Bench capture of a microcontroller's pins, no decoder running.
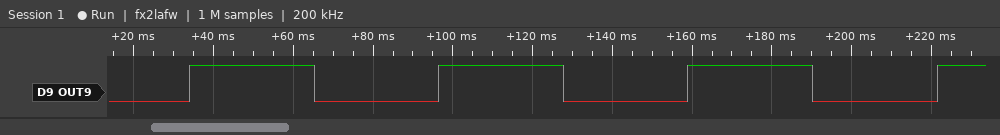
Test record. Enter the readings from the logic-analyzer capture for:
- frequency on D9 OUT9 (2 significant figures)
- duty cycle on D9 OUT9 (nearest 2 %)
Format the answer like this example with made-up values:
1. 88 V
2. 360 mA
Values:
1. 16 Hz
2. 50 %
